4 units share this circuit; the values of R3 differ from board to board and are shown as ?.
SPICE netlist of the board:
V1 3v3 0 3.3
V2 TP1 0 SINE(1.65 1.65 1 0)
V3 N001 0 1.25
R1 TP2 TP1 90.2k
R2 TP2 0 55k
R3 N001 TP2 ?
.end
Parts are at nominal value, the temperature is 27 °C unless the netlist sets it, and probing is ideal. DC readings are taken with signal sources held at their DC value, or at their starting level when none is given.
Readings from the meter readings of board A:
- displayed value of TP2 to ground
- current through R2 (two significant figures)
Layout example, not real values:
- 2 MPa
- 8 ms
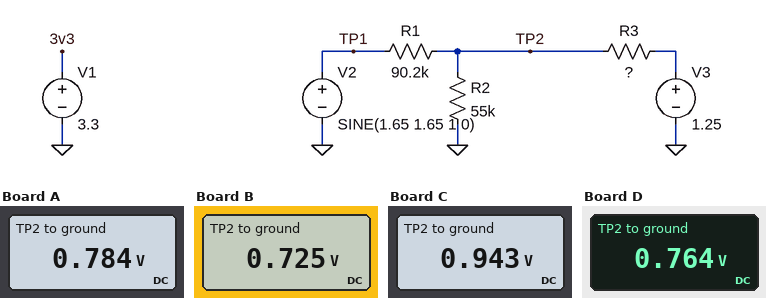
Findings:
- 0.784 V
- 14 µA
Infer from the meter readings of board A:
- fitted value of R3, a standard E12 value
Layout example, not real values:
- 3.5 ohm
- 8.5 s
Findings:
- 100 kΩ
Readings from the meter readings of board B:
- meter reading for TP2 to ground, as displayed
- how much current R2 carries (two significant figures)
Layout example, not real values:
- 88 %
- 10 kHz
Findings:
- 0.725 V
- 13 µA
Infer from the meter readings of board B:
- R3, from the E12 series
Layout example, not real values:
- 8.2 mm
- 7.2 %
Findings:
- 180 kΩ
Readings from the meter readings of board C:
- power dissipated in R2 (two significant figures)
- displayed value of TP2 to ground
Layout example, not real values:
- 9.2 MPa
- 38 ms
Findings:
- 16 µW
- 0.943 V
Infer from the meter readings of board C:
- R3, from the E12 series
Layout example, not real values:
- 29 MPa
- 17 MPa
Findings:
- 33 kΩ
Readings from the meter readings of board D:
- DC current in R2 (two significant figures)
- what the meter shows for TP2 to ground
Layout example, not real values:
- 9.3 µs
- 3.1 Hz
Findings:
- 14 µA
- 0.764 V
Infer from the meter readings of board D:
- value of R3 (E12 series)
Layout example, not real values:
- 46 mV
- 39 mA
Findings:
- 120 kΩ
